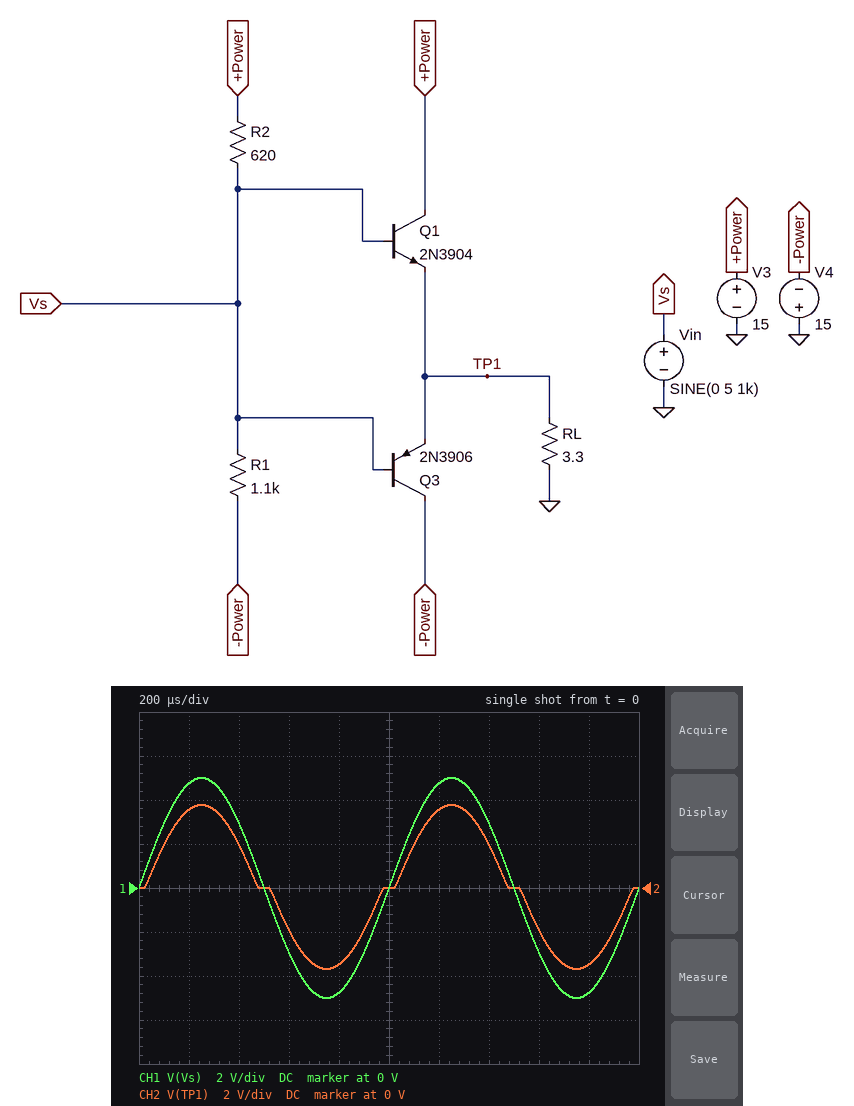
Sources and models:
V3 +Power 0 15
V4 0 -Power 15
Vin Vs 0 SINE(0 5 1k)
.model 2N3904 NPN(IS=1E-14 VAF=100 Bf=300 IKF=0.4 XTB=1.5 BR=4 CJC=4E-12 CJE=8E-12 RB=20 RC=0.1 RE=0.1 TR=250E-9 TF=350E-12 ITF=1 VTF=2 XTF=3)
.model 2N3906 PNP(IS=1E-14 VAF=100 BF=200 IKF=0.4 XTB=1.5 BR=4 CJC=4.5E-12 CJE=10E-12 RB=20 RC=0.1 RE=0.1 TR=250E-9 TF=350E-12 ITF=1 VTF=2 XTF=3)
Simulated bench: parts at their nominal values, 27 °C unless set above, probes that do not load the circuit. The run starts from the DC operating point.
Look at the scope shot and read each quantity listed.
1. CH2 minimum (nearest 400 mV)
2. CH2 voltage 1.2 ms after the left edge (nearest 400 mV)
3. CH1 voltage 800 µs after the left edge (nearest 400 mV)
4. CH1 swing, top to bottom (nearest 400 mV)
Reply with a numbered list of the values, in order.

1. -3.6 V
2. 3.6 V
3. -4.8 V
4. 10.0 V
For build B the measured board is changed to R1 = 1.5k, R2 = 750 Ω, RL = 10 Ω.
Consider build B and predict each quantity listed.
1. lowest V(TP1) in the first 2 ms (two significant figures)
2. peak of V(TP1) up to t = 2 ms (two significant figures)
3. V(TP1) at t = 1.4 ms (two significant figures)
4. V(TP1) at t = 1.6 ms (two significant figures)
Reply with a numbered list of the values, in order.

1. -4.1 V
2. 4.1 V
3. 2.1 V
4. -2.1 V
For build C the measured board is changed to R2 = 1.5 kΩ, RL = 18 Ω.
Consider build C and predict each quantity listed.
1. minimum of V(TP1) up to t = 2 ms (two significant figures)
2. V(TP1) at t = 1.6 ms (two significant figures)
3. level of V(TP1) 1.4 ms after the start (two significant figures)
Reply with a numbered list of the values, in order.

1. -4.1 V
2. -2.1 V
3. 2.1 V
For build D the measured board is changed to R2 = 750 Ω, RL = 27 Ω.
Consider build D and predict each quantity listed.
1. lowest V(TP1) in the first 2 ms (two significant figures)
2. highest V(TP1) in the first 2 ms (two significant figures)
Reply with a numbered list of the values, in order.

1. -4.2 V
2. 4.2 V
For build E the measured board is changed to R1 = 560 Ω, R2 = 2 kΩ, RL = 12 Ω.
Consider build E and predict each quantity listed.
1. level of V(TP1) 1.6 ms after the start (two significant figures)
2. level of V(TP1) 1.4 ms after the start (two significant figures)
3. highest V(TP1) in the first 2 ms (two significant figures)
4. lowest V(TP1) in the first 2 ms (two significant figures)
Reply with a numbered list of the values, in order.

1. -2.1 V
2. 2.1 V
3. 4.1 V
4. -4.1 V
